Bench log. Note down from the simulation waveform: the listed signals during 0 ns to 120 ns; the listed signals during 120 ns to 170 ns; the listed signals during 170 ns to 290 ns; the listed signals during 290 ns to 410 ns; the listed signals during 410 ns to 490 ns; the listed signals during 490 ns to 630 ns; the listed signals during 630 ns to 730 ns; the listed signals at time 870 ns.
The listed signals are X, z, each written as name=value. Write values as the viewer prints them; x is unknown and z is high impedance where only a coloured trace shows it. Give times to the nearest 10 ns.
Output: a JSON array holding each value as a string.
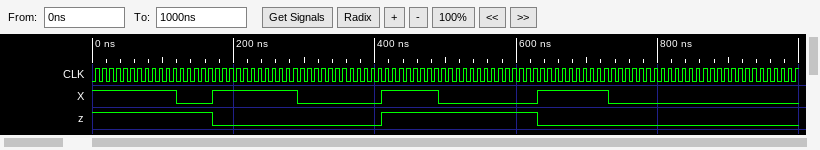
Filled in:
["X=1, z=1", "X=0, z=1", "X=1, z=0", "X=0, z=0", "X=1, z=1", "X=0, z=1", "X=1, z=0", "X=0, z=0"]
